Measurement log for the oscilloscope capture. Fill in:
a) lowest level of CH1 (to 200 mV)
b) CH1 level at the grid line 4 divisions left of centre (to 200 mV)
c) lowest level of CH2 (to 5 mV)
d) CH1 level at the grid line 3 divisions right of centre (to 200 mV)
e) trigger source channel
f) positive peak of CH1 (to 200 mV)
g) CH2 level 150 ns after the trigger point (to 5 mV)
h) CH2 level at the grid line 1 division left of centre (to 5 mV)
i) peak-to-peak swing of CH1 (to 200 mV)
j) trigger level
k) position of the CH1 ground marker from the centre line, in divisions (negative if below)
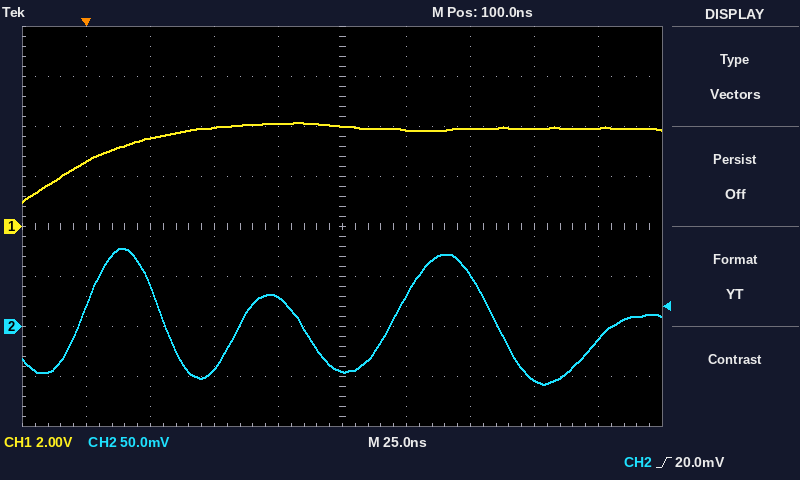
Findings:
1.0 V
2.6 V
-60 mV
4.0 V
CH2
4.2 V
50 mV
30 mV
3.2 V
20.0 mV
0.0 div
